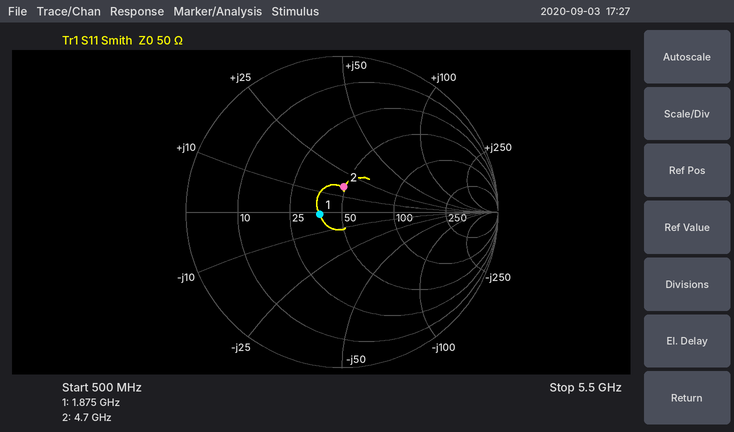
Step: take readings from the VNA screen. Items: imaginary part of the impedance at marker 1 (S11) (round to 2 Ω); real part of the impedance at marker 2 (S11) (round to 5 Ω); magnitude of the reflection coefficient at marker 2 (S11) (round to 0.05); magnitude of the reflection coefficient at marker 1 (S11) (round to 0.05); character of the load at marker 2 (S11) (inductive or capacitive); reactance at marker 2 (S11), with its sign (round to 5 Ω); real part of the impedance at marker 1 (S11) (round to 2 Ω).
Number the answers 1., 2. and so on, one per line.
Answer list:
1. -2 Ω
2. 50 Ω
3. 0.15
4. 0.15
5. inductive
6. +15 Ω
7. 38 Ω
